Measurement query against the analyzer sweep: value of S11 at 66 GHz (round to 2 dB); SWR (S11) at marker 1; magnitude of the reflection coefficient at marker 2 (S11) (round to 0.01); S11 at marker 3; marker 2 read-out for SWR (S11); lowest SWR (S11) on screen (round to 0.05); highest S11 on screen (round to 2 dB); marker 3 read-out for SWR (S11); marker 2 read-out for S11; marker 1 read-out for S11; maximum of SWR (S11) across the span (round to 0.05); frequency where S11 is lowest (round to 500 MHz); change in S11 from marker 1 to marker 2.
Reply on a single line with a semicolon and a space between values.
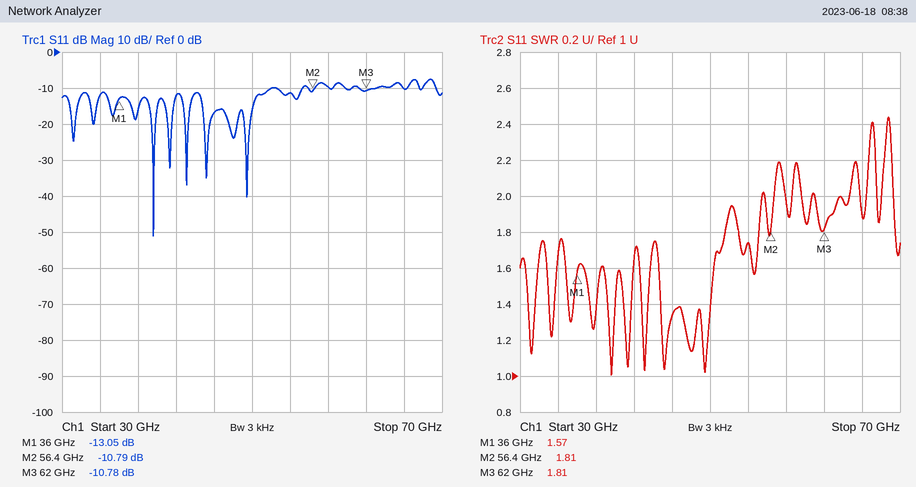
-10 dB; 1.57; 0.29; -10.78 dB; 1.81; 1.00; -8 dB; 1.81; -10.79 dB; -13.05 dB; 2.45; 39.5 GHz; 2.26 dB
